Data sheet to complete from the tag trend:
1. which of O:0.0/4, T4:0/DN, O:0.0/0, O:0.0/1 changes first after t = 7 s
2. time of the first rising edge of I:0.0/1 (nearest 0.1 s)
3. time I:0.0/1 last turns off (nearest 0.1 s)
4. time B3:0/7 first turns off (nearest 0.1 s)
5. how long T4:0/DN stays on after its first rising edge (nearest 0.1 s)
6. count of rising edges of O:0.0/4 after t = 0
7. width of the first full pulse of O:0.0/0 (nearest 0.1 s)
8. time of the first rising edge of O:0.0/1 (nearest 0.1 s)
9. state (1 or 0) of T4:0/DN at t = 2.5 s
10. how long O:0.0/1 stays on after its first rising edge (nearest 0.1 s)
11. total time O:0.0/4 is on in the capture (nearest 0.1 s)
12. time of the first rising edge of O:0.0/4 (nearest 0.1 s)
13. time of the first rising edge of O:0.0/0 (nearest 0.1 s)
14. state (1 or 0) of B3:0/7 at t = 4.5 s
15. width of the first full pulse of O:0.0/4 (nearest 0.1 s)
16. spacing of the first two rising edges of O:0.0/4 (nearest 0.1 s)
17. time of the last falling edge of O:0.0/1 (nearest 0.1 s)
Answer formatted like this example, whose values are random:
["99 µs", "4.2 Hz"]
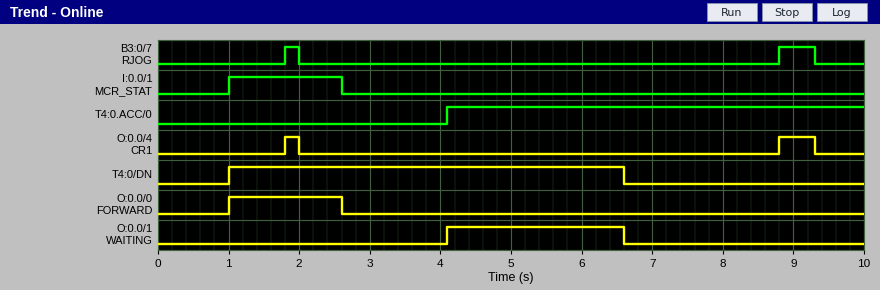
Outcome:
["O:0.0/4", "1.0 s", "2.6 s", "2.0 s", "5.6 s", "2", "1.6 s", "4.1 s", "1", "2.5 s", "0.7 s", "1.8 s", "1.0 s", "0", "0.2 s", "7.0 s", "6.6 s"]
